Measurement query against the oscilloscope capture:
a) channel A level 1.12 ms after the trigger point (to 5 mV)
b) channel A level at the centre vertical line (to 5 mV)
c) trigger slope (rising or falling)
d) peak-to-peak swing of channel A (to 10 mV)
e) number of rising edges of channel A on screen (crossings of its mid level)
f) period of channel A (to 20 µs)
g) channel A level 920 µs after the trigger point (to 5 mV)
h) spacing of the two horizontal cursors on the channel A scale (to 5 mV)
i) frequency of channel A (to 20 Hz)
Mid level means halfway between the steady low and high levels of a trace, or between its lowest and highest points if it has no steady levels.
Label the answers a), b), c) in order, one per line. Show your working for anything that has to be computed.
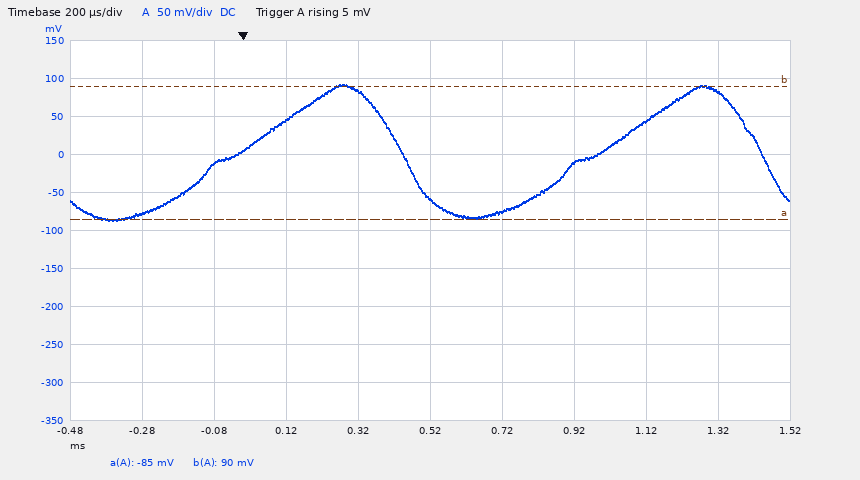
a) 45 mV
b) -60 mV
c) rising
d) 180 mV
e) 2
f) 1.00 ms
g) -10 mV
h) 175 mV
i) 1 / 1.00 ms ≈ 1.00 kHz
